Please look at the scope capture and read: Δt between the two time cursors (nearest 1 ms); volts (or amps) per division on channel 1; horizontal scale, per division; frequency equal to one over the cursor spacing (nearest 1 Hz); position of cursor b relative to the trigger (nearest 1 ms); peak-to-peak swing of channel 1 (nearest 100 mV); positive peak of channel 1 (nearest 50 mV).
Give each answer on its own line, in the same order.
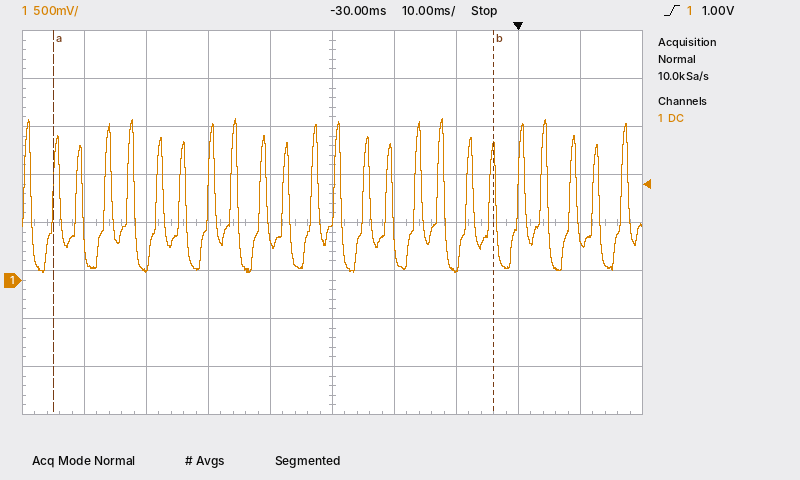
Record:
71 ms
500 mV
10 ms
14 Hz
-4 ms
1.60 V
1.70 V
